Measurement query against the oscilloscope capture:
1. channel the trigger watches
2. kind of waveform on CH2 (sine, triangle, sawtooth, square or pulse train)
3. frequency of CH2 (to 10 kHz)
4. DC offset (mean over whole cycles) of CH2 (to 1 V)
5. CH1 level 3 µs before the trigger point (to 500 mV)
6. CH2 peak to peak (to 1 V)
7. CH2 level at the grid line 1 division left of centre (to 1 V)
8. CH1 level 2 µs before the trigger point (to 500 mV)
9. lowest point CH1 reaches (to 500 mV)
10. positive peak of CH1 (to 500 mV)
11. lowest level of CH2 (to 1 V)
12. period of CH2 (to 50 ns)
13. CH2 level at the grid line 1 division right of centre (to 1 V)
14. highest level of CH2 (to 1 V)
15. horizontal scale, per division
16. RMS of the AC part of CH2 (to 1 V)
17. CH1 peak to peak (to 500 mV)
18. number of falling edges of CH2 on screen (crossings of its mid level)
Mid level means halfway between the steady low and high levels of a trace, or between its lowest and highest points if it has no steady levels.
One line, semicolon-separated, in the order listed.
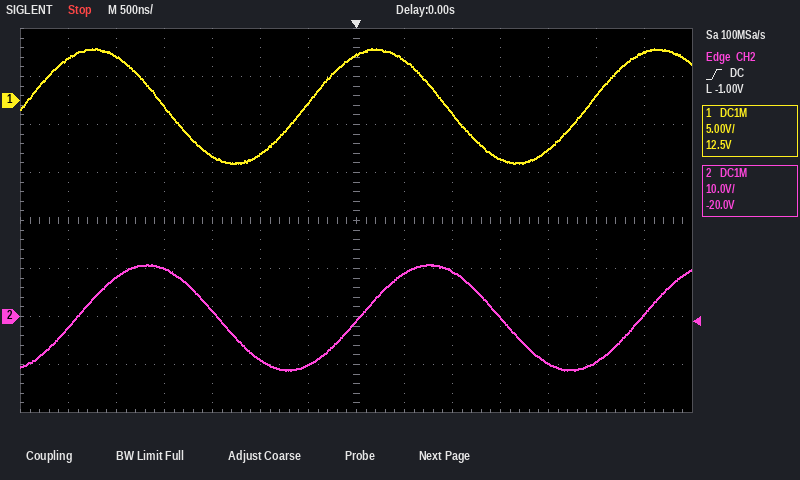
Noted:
CH2; sine; 340 kHz; 0 V; 4.5 V; 22 V; -10 V; -500 mV; -6.5 V; 5.5 V; -11 V; 2.95 µs; 9 V; 11 V; 500 ns; 8 V; 12.0 V; 2
